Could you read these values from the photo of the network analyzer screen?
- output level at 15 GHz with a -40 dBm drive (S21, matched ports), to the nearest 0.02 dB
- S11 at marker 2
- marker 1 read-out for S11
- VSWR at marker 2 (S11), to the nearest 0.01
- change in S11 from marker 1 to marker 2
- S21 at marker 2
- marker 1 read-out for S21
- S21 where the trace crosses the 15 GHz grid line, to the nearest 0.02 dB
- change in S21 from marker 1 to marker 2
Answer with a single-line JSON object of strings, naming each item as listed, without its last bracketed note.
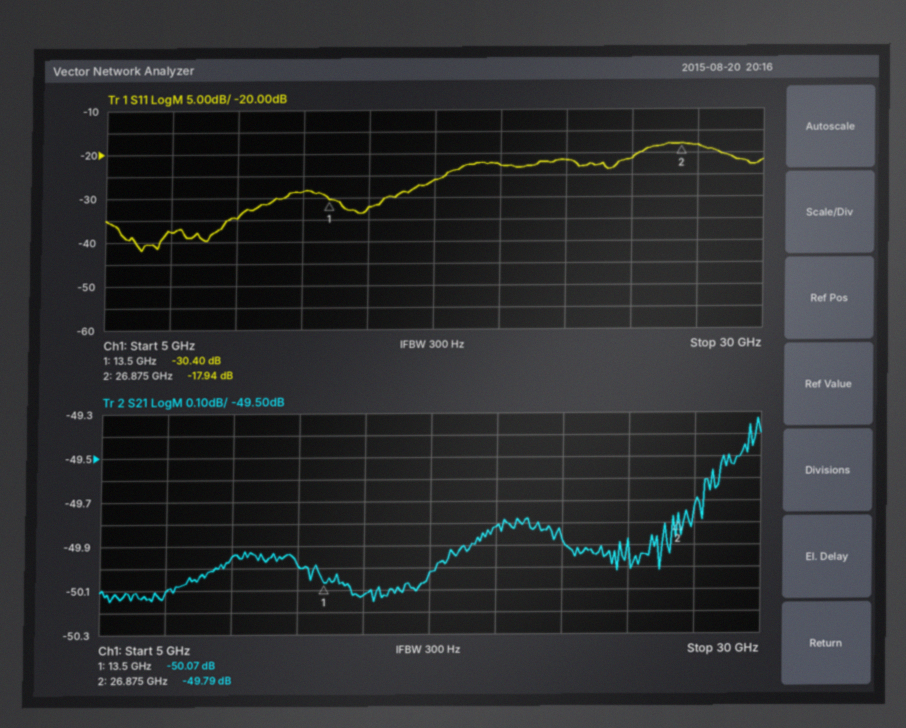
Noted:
{"output level at 15 GHz with a -40 dBm drive (S21, matched ports), to the nearest 0.02 dB": "-90.12 dBm", "S11 at marker 2": "-17.94 dB", "marker 1 read-out for S11": "-30.40 dB", "VSWR at marker 2 (S11), to the nearest 0.01": "1.29", "change in S11 from marker 1 to marker 2": "12.46 dB", "S21 at marker 2": "-49.79 dB", "marker 1 read-out for S21": "-50.07 dB", "S21 where the trace crosses the 15 GHz grid line, to the nearest 0.02 dB": "-50.12 dB", "change in S21 from marker 1 to marker 2": "0.28 dB"}
